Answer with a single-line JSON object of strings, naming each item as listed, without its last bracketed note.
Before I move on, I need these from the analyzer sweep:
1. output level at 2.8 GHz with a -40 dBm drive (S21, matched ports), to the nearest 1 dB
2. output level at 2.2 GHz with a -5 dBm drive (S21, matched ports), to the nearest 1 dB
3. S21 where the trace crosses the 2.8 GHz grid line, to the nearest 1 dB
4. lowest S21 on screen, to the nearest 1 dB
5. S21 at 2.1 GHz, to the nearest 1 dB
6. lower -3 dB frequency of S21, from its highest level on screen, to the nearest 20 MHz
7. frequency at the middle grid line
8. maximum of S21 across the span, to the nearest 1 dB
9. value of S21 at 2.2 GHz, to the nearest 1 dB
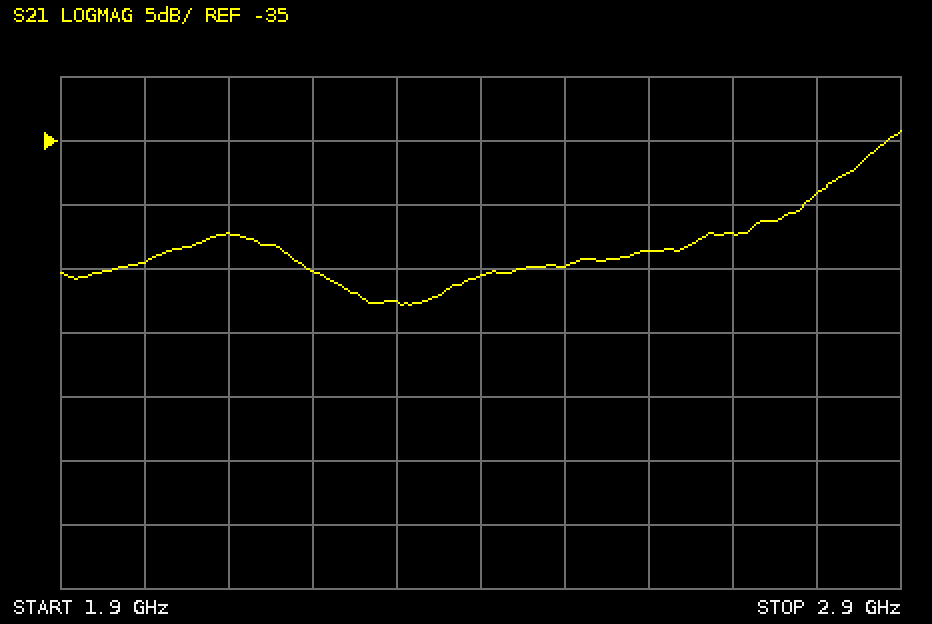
{"output level at 2.8 GHz with a -40 dBm drive (S21, matched ports), to the nearest 1 dB": "-79 dBm", "output level at 2.2 GHz with a -5 dBm drive (S21, matched ports), to the nearest 1 dB": "-50 dBm", "S21 where the trace crosses the 2.8 GHz grid line, to the nearest 1 dB": "-39 dB", "lowest S21 on screen, to the nearest 1 dB": "-48 dB", "S21 at 2.1 GHz, to the nearest 1 dB": "-42 dB", "lower -3 dB frequency of S21, from its highest level on screen, to the nearest 20 MHz": "2.84 GHz", "frequency at the middle grid line": "2.4 GHz", "maximum of S21 across the span, to the nearest 1 dB": "-34 dB", "value of S21 at 2.2 GHz, to the nearest 1 dB": "-45 dB"}
